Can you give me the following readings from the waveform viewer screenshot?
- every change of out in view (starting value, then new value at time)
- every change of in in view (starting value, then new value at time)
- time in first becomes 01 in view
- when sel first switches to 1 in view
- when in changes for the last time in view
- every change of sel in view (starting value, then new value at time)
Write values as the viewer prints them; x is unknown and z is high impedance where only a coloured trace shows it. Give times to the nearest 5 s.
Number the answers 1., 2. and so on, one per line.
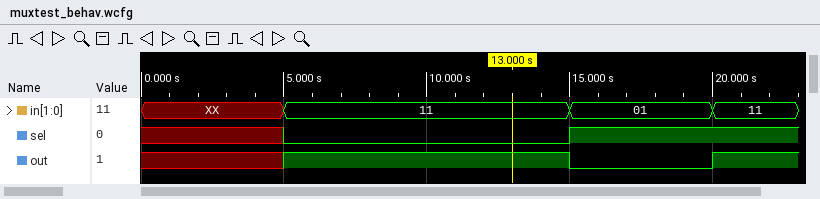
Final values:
1. x, 1 at 5 s, 0 at 15 s, 1 at 20 s
2. XX, 11 at 5 s, 01 at 15 s, 11 at 20 s
3. 15 s
4. 15 s
5. 20 s
6. x, 0 at 5 s, 1 at 15 s
